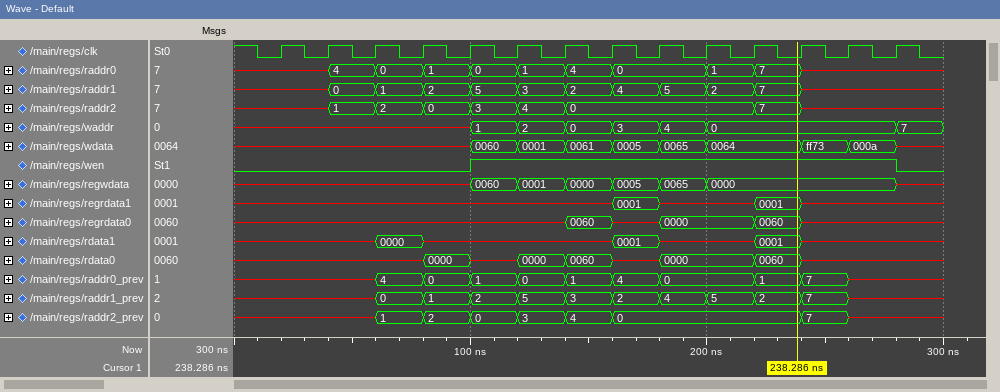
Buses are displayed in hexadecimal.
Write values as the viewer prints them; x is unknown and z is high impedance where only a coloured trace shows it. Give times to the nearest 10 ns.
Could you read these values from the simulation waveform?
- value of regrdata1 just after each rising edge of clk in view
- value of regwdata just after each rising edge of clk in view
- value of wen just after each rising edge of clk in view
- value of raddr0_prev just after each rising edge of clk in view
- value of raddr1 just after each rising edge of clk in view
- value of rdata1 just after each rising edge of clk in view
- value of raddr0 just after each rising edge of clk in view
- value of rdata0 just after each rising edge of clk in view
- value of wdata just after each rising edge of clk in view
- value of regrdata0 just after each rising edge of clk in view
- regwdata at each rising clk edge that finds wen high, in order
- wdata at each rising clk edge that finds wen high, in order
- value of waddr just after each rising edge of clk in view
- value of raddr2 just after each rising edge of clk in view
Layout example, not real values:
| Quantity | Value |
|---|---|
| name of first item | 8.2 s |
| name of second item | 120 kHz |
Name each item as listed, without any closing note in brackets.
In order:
| Quantity | Value |
|---|---|
| value of regrdata1 just after each rising edge of clk in view | x, x, x, x, x, x, x, 0001, x, x, 0001, x, x, x |
| value of regwdata just after each rising edge of clk in view | x, x, x, x, 0060, 0001, 0000, 0005, 0065, 0000, 0000, 0000, 0000, x |
| value of wen just after each rising edge of clk in view | 0 0 0 0 1 1 1 1 1 1 1 1 1 0 |
| value of raddr0_prev just after each rising edge of clk in view | x, x, 4, 0, 1, 0, 1, 4, 0, 0, 1, 7, x, x |
| value of raddr1 just after each rising edge of clk in view | x, 0, 1, 2, 5, 3, 2, 4, 5, 2, 7, x, x, x |
| value of rdata1 just after each rising edge of clk in view | x, x, 0000, x, x, x, x, 0001, x, x, 0001, x, x, x |
| value of raddr0 just after each rising edge of clk in view | x, 4, 0, 1, 0, 1, 4, 0, 0, 1, 7, x, x, x |
| value of rdata0 just after each rising edge of clk in view | x, x, x, 0000, x, 0000, 0060, x, 0000, 0000, 0060, x, x, x |
| value of wdata just after each rising edge of clk in view | x, x, x, x, 0060, 0001, 0061, 0005, 0065, 0064, 0064, ff73, 000a, x |
| value of regrdata0 just after each rising edge of clk in view | x, x, x, x, x, x, 0060, x, 0000, 0000, 0060, x, x, x |
| regwdata at each rising clk edge that finds wen high, in order | 0060, 0001, 0000, 0005, 0065, 0000, 0000, 0000, 0000 |
| wdata at each rising clk edge that finds wen high, in order | 0060, 0001, 0061, 0005, 0065, 0064, 0064, ff73, 000a |
| value of waddr just after each rising edge of clk in view | x, x, x, x, 1, 2, 0, 3, 4, 0, 0, 0, 0, 7 |
| value of raddr2 just after each rising edge of clk in view | x, 1, 2, 0, 3, 4, 0, 0, 0, 0, 7, x, x, x |
